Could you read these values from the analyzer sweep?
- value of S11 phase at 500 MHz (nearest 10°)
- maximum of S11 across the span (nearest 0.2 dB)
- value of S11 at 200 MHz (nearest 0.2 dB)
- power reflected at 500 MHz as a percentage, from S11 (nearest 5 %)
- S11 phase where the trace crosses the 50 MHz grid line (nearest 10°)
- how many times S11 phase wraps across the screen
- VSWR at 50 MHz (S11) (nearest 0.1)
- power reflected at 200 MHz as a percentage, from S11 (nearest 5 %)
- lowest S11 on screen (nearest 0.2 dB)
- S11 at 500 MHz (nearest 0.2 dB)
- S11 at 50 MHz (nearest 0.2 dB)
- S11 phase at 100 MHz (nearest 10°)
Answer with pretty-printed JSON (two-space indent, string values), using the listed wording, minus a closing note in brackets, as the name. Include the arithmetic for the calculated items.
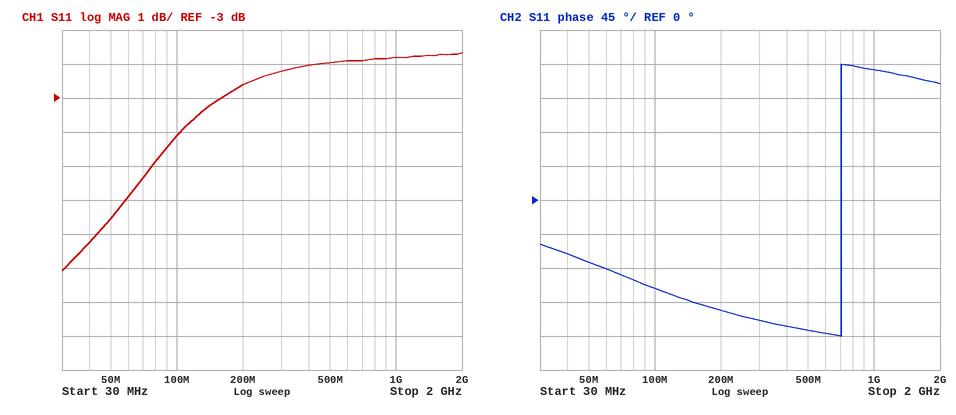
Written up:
{
  "value of S11 phase at 500 MHz": "-170°",
  "maximum of S11 across the span": "-1.6 dB",
  "value of S11 at 200 MHz": "-2.6 dB",
  "power reflected at 500 MHz as a percentage, from S11": "10^(-2/10) ≈ 63.1 %, so 65 % to the nearest 5 %",
  "S11 phase where the trace crosses the 50 MHz grid line": "-80°",
  "how many times S11 phase wraps across the screen": "1",
  "VSWR at 50 MHz (S11)": "|Γ| = 10^(-6.6/20) = 0.4677; VSWR = (1 + 0.4677)/(1 − 0.4677) ≈ 2.8",
  "power reflected at 200 MHz as a percentage, from S11": "10^(-2.6/10) ≈ 55 %",
  "lowest S11 on screen": "-8.0 dB",
  "S11 at 500 MHz": "-2.0 dB",
  "S11 at 50 MHz": "-6.6 dB",
  "S11 phase at 100 MHz": "-120°"
}
